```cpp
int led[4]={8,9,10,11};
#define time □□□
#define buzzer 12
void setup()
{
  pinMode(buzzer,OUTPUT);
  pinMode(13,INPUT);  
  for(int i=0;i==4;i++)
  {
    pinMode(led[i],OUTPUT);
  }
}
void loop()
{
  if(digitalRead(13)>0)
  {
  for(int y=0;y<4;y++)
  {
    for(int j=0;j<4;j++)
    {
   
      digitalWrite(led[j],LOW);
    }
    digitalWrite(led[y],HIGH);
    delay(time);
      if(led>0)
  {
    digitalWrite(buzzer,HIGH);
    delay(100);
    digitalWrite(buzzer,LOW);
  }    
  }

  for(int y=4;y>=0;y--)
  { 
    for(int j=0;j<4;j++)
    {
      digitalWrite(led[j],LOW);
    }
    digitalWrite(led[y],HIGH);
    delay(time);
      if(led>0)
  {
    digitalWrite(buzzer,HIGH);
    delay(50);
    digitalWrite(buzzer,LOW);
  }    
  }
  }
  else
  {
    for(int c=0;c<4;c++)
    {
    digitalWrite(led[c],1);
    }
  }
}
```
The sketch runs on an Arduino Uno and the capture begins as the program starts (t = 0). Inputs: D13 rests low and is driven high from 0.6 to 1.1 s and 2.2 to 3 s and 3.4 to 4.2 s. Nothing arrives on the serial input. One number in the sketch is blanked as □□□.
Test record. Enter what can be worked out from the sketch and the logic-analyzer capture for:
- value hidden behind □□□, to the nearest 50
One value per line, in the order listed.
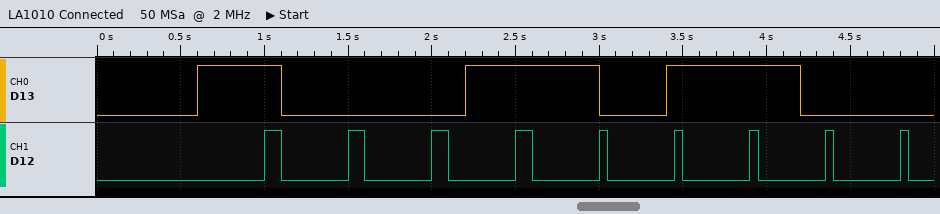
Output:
400
